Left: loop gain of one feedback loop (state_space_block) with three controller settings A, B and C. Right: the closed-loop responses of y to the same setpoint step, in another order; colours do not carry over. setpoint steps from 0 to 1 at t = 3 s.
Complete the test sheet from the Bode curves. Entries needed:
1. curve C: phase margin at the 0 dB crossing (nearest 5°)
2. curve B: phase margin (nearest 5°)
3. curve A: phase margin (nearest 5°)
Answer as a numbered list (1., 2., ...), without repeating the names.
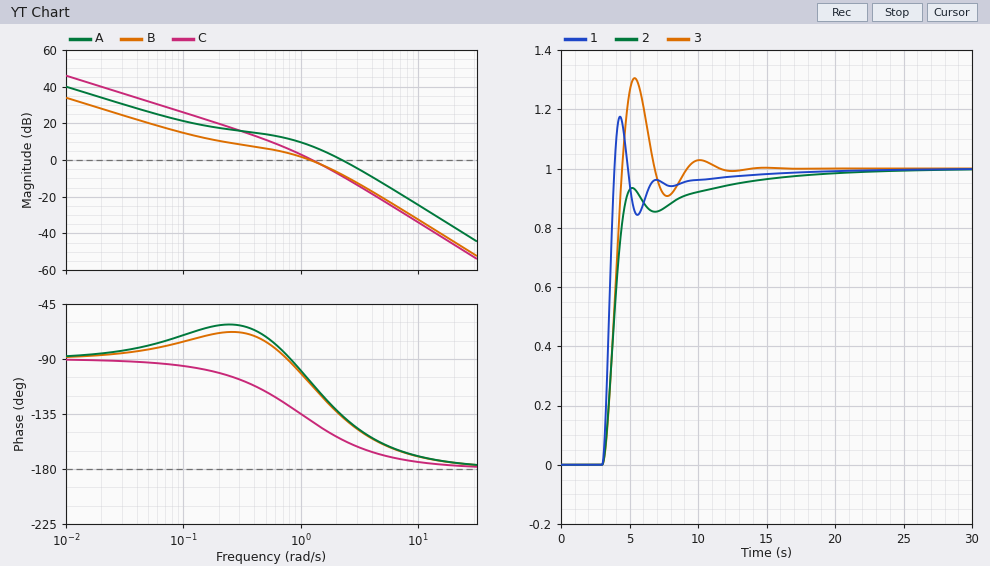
1. 40°
2. 70°
3. 45°
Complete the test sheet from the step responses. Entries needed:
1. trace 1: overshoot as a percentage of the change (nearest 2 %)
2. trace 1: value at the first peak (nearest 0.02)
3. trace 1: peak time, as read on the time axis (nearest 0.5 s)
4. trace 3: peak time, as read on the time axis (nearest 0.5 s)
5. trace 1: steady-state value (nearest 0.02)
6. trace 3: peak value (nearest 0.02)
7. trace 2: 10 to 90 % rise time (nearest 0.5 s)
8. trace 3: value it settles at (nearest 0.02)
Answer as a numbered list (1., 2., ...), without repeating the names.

1. 18 %
2. 1.18
3. 4.5 s
4. 5.5 s
5. 1.00
6. 1.30
7. 1.5 s
8. 1.00
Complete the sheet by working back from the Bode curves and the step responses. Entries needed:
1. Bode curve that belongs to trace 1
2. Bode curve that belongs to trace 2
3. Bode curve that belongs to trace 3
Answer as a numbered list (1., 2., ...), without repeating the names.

1. A
2. B
3. C
